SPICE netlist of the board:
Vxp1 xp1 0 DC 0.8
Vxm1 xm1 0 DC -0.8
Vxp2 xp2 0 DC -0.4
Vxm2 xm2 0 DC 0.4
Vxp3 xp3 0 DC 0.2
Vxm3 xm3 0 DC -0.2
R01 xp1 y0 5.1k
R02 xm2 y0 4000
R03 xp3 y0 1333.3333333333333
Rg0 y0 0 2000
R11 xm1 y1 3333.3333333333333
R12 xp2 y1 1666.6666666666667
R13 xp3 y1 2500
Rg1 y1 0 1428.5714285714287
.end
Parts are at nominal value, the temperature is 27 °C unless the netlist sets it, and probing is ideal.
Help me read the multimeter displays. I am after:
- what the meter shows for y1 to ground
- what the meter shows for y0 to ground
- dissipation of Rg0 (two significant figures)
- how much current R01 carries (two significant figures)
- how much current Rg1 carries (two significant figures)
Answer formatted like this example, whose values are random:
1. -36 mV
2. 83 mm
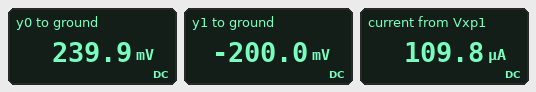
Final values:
1. -200.0 mV
2. 239.9 mV
3. 29 µW
4. 110 µA
5. 140 µA
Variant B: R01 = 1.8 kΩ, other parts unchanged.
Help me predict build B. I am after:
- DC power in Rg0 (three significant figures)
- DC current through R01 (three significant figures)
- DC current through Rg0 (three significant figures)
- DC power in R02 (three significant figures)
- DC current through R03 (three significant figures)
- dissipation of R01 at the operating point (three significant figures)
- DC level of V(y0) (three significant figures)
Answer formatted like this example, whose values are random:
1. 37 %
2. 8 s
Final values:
1. 57.1 µW
2. 257 µA
3. 169 µA
4. 966 nW
5. 103 µA
6. 119 µW
7. 338 mV
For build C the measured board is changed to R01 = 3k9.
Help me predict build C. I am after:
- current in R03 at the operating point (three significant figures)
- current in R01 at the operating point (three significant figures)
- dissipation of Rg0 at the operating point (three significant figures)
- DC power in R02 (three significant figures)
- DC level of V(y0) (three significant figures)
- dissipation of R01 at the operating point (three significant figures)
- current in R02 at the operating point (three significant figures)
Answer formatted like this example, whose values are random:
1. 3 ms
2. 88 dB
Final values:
1. 44.3 µA
2. 139 µA
3. 33.6 µW
4. 4.96 µW
5. 259 mV
6. 75.0 µW
7. 35.2 µA
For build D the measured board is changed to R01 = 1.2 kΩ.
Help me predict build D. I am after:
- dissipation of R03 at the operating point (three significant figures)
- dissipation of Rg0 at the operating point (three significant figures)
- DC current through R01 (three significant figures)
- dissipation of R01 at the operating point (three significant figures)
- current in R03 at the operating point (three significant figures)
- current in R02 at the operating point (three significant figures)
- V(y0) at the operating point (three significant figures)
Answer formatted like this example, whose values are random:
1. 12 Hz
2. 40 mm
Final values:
1. 27.9 µW
2. 77.2 µW
3. 339 µA
4. 138 µW
5. 145 µA
6. 1.79 µA
7. 393 mV
